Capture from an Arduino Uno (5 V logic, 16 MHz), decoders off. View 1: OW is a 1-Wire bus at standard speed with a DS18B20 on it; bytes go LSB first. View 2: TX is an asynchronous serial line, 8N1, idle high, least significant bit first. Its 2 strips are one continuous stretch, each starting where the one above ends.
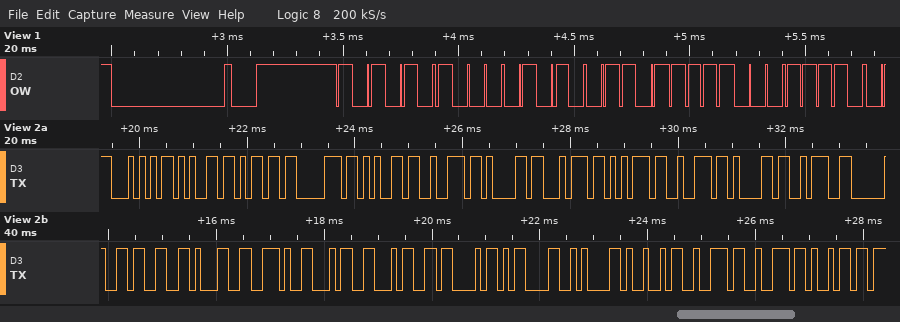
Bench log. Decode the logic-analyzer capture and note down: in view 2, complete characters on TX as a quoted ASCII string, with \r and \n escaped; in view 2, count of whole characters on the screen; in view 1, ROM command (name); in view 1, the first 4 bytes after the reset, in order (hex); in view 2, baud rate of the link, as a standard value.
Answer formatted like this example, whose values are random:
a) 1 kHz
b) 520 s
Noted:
a) "Temperatura: 31.44C\r\nIrri"
b) 25
c) Match ROM
d) 55 28 FB 78
e) 9600 baud
